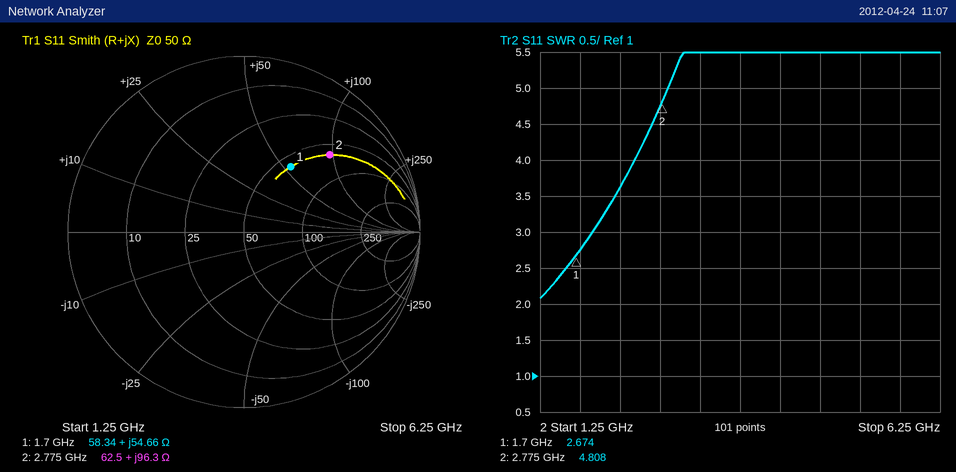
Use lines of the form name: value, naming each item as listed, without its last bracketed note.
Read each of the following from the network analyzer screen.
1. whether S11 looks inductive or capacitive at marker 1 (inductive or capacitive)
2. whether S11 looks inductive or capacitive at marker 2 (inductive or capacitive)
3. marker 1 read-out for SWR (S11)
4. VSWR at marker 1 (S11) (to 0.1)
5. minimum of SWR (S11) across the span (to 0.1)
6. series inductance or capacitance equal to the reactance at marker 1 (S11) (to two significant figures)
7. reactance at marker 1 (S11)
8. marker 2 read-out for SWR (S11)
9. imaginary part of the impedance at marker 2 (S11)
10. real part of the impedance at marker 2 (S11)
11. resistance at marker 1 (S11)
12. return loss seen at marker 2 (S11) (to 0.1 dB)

whether S11 looks inductive or capacitive at marker 1: inductive
whether S11 looks inductive or capacitive at marker 2: inductive
marker 1 read-out for SWR: 2.674
VSWR at marker 1 (S11): 2.7
minimum of SWR (S11) across the span: 2.1
series inductance or capacitance equal to the reactance at marker 1 (S11): 5.1 nH
reactance at marker 1: +54.66 Ω
marker 2 read-out for SWR: 4.808
imaginary part of the impedance at marker 2: +96.3 Ω
real part of the impedance at marker 2: 62.5 Ω
resistance at marker 1: 58.34 Ω
return loss seen at marker 2 (S11): 3.7 dB
